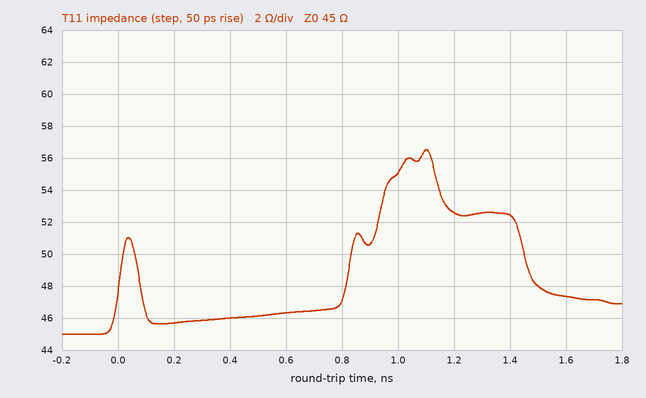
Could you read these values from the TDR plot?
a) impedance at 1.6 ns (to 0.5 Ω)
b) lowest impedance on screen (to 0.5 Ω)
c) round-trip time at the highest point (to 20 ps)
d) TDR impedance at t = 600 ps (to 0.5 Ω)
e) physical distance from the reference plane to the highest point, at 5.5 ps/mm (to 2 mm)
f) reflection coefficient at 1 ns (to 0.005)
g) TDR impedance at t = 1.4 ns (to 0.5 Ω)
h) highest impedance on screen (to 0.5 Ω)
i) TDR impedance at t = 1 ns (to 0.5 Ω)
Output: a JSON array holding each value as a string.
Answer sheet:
["47.5 Ω", "45.0 Ω", "1.10 ns", "46.5 Ω", "100 mm", "+0.100", "52.5 Ω", "56.5 Ω", "55.0 Ω"]
